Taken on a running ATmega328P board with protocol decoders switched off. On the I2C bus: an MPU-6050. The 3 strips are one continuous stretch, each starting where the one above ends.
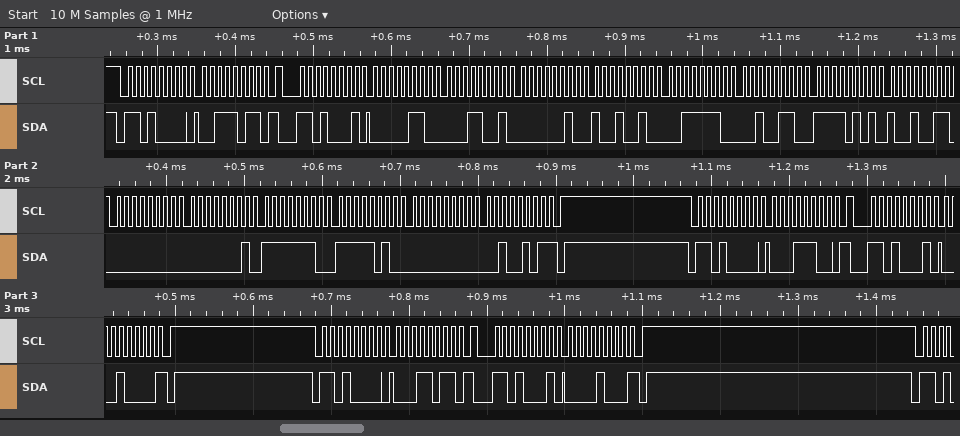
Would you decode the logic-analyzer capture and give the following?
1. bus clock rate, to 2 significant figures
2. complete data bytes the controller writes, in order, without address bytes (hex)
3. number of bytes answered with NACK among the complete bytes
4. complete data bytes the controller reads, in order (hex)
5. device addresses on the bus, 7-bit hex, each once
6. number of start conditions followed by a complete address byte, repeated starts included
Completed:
100 kHz
3B 1C 1B
3
06 19 02 92 3E 26 F5 93 00 01 FE FA 00 25 10 08
0x68
6
